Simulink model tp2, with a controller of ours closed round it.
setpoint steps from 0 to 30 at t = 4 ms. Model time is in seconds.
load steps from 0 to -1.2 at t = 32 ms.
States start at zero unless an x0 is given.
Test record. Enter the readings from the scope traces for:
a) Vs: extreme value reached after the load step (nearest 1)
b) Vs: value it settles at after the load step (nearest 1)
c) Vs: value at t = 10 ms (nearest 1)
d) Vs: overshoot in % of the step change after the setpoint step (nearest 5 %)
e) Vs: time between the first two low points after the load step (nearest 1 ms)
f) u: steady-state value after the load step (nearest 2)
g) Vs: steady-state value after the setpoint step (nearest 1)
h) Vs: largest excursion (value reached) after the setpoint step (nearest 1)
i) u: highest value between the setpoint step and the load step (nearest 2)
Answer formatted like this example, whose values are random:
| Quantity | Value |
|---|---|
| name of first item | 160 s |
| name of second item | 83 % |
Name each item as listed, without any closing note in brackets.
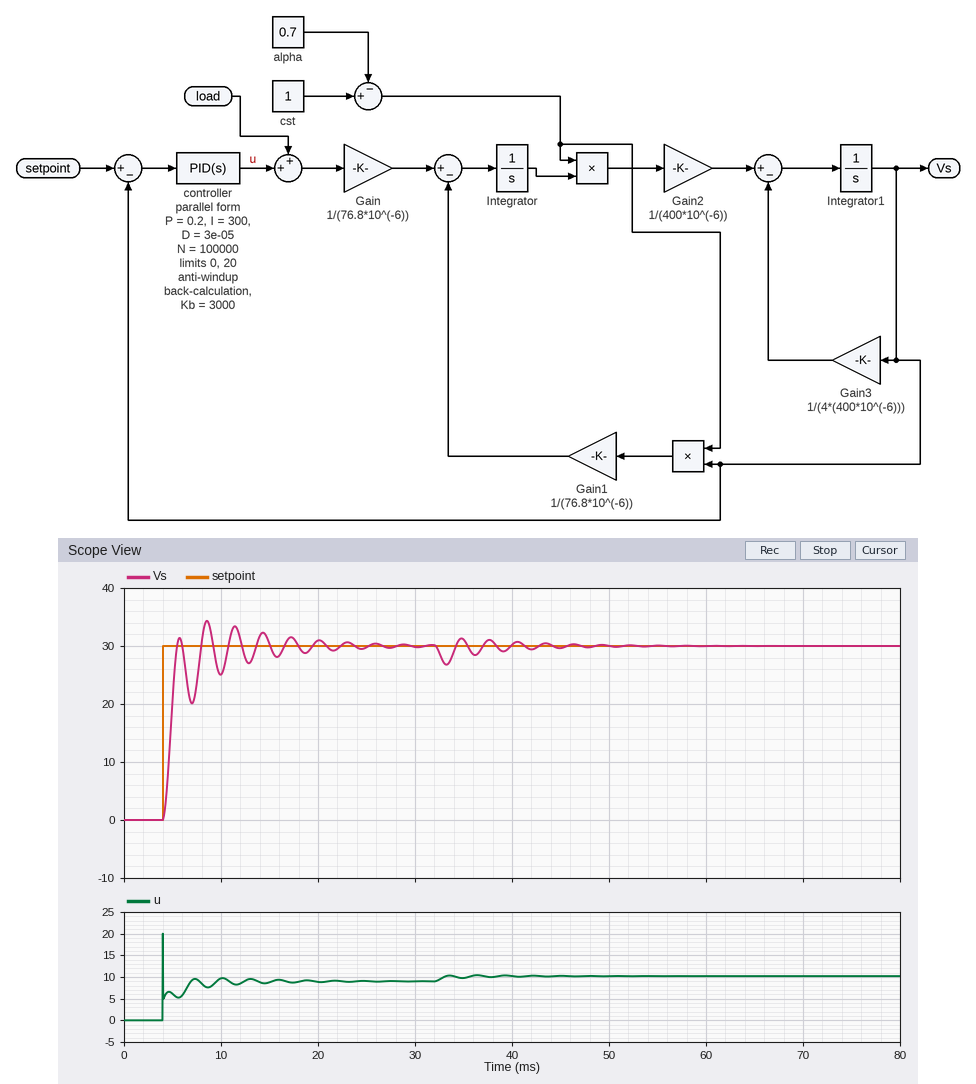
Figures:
| Quantity | Value |
|---|---|
| Vs: extreme value reached after the load step | 27 |
| Vs: value it settles at after the load step | 30 |
| Vs: value at t = 10 ms | 25 |
| Vs: overshoot in % of the step change after the setpoint step | 15 % |
| Vs: time between the first two low points after the load step | 3 ms |
| u: steady-state value after the load step | 10 |
| Vs: steady-state value after the setpoint step | 30 |
| Vs: largest excursion (value reached) after the setpoint step | 34 |
| u: highest value between the setpoint step and the load step | 20 |
